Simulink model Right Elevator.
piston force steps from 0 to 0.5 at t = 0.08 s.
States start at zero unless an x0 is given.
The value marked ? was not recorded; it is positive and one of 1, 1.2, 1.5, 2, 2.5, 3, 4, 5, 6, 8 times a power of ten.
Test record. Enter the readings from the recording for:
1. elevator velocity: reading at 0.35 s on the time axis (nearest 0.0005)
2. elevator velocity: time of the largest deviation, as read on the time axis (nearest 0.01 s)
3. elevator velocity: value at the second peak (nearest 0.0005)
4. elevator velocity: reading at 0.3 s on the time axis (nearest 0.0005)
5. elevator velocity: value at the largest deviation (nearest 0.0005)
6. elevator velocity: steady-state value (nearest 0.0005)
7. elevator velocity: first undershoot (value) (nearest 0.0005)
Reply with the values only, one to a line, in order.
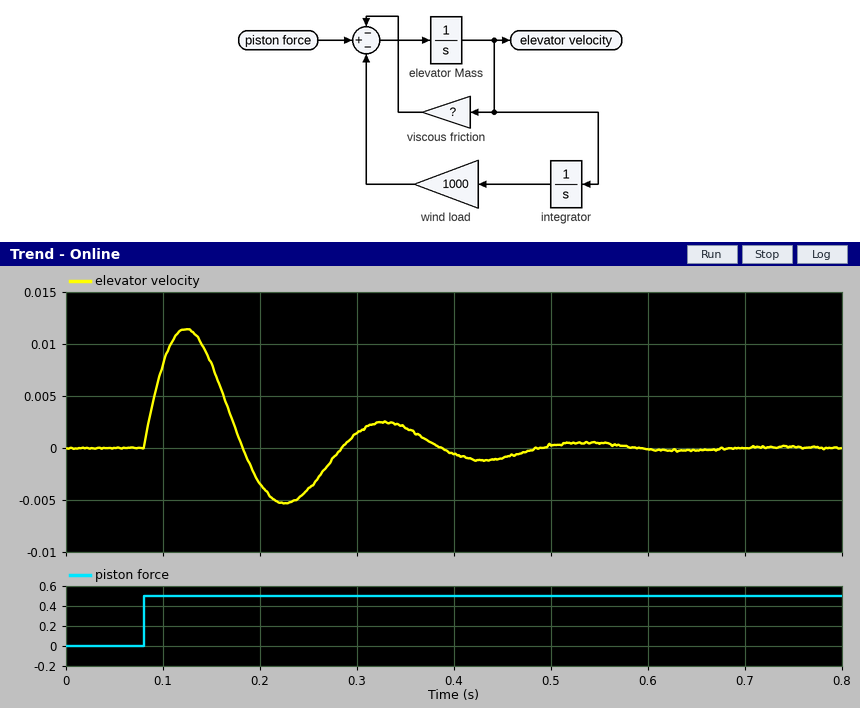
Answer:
0.0020
0.12 s
0.0025
0.0015
0.0115
0.0000
-0.0055
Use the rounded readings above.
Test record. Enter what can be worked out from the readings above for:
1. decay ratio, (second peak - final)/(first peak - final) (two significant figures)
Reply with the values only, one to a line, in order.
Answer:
0.22
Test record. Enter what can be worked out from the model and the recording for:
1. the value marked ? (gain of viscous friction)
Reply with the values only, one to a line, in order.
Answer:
15
